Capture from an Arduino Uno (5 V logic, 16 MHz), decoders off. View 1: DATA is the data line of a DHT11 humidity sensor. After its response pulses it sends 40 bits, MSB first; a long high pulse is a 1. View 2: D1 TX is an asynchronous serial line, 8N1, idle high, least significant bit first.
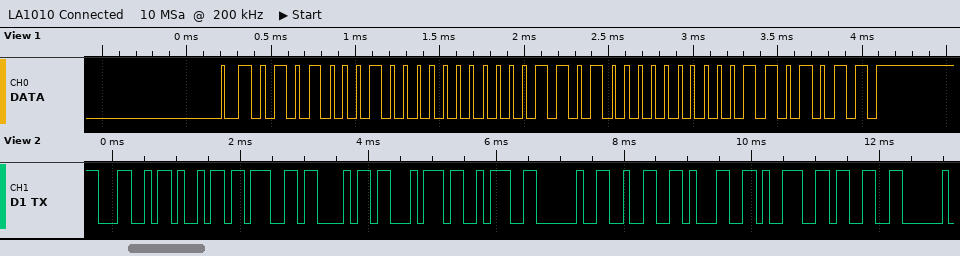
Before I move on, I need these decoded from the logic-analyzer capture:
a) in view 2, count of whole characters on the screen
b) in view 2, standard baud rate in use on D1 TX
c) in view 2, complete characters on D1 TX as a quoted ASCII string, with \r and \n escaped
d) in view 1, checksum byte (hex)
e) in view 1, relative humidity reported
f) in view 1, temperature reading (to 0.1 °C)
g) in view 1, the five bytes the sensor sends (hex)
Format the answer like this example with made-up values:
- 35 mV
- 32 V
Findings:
- 11
- 9600 baud
- "Light: 2193"
- 0x6B
- 81 %
- 26.0 °C
- 51 00 1A 00 6B
